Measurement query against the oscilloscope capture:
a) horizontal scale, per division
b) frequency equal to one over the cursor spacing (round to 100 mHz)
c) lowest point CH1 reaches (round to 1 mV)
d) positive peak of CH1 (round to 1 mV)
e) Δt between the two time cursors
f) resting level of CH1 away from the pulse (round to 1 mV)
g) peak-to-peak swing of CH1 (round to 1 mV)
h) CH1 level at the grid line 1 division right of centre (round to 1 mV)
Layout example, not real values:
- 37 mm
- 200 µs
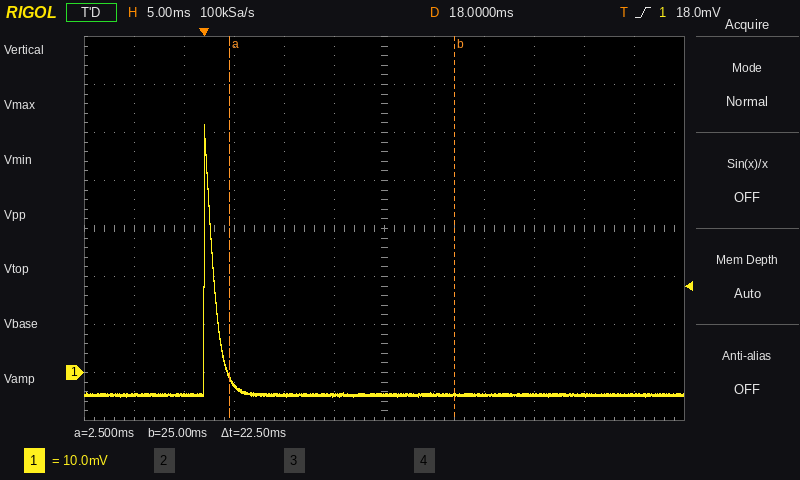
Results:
- 5 ms
- 44.4 Hz
- -5 mV
- 52 mV
- 22.5 ms
- -5 mV
- 57 mV
- -5 mV
